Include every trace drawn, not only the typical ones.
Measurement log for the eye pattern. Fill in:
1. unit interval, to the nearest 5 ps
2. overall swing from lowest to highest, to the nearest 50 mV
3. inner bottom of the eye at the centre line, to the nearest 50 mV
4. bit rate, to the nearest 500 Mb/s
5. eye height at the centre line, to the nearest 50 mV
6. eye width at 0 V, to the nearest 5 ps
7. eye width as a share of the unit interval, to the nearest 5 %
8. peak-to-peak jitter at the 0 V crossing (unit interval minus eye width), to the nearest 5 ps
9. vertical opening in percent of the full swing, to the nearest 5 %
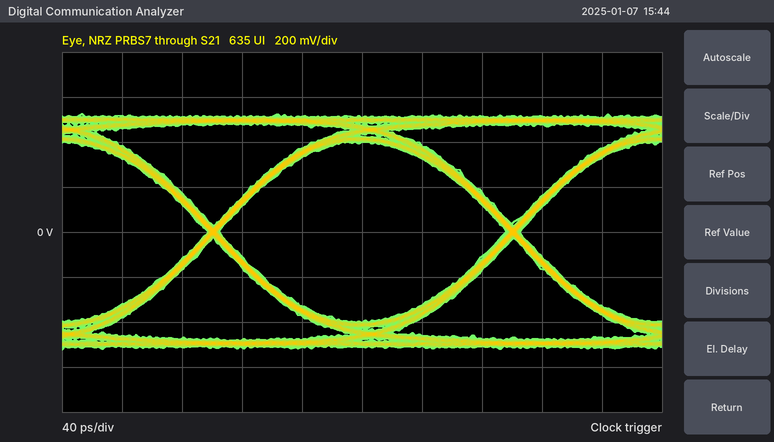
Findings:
200 ps
1.05 V
-400 mV
5.0 Gb/s
800 mV
190 ps
95 %
10 ps
75 %
